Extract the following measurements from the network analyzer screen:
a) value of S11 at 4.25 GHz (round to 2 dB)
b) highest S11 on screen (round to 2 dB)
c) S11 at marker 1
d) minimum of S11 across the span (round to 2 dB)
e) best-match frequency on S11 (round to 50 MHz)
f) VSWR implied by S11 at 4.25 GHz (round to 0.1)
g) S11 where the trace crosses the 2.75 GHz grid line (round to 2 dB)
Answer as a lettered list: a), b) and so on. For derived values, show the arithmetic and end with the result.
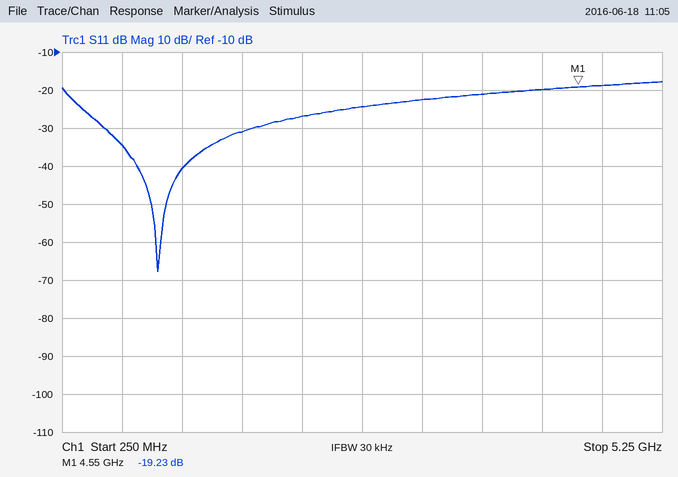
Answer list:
a) -20 dB
b) -18 dB
c) -19.23 dB
d) -68 dB
e) 1.05 GHz
f) |Γ| = 10^(-20/20) = 0.1000; VSWR = (1 + 0.1000)/(1 − 0.1000) ≈ 1.2
g) -24 dB
